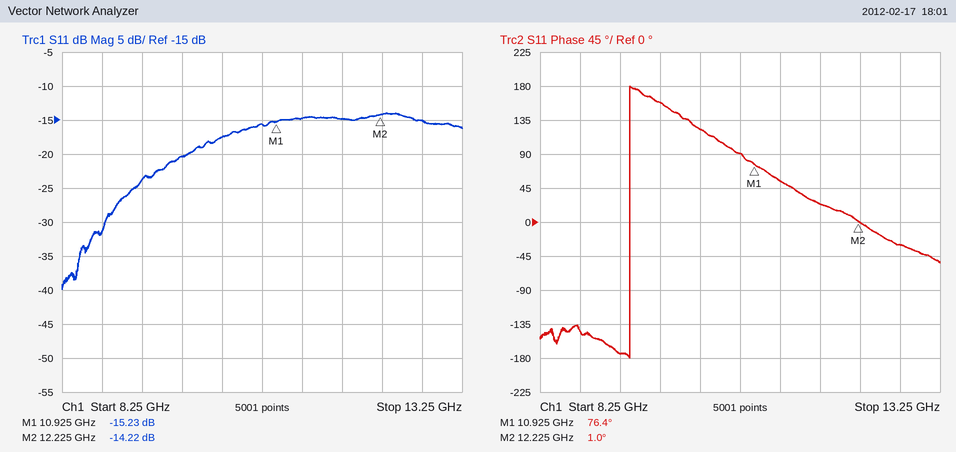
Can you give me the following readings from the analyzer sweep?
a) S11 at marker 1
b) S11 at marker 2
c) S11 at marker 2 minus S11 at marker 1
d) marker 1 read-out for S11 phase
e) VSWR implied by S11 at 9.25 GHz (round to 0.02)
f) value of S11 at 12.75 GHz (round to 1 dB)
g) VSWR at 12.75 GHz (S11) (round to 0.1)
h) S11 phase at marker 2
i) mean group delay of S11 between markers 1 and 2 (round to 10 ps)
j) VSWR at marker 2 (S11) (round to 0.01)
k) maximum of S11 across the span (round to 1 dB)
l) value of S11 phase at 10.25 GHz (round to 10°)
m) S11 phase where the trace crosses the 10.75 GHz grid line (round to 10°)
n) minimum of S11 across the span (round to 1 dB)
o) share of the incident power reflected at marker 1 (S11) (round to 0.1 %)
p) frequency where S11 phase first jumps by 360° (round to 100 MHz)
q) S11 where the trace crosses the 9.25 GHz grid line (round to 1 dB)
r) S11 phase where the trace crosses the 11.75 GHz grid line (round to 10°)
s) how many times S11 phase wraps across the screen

-15.23 dB
-14.22 dB
1.01 dB
76.4°
1.14
-15 dB
1.4
1.0°
160 ps
1.48
-14 dB
120°
90°
-40 dB
3.0 %
9.4 GHz
-24 dB
20°
1
